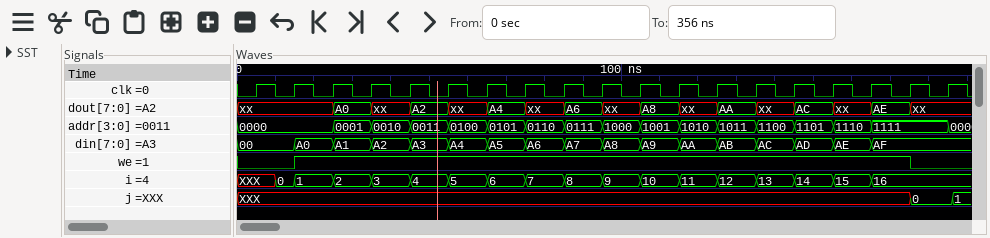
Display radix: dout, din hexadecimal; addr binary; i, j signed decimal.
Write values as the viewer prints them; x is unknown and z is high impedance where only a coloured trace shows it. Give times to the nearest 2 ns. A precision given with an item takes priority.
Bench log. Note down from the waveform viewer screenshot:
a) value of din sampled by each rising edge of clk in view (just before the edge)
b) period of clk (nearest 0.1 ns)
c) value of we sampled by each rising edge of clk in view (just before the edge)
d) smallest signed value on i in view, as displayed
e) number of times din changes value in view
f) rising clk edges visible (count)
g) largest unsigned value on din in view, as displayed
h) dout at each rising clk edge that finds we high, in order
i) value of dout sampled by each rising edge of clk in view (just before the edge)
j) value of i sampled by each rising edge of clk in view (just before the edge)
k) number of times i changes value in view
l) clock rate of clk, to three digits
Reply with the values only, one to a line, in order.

00, 00, A0, A1, A2, A3, A4, A5, A6, A7, A8, A9, AA, AB, AC, AD, AE, AF, AF
10 ns
0 0 1 1 1 1 1 1 1 1 1 1 1 1 1 1 1 1 0
0
16
19
AF
xx, A0, xx, A2, xx, A4, xx, A6, xx, A8, xx, AA, xx, AC, xx, AE
xx, xx, xx, A0, xx, A2, xx, A4, xx, A6, xx, A8, xx, AA, xx, AC, xx, AE, xx
XXX, 0, 1, 2, 3, 4, 5, 6, 7, 8, 9, 10, 11, 12, 13, 14, 15, 16, 16
17
100 MHz
